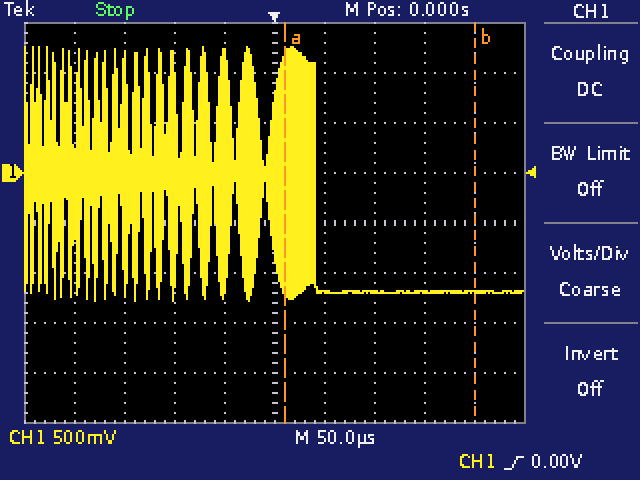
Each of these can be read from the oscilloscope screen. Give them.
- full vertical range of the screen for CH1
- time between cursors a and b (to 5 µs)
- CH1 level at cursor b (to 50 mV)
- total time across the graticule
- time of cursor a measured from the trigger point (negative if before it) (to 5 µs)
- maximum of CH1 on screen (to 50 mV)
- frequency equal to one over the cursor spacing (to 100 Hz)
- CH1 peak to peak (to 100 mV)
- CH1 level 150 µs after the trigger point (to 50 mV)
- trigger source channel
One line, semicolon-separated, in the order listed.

4 V; 190 µs; -1.20 V; 500 µs; +10 µs; 1.25 V; 5.3 kHz; 2.50 V; -1.20 V; CH1
